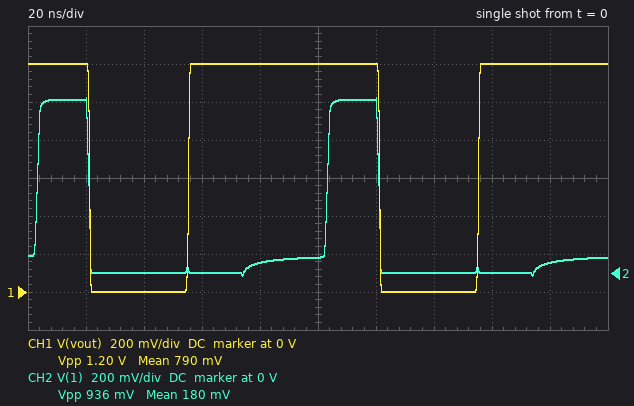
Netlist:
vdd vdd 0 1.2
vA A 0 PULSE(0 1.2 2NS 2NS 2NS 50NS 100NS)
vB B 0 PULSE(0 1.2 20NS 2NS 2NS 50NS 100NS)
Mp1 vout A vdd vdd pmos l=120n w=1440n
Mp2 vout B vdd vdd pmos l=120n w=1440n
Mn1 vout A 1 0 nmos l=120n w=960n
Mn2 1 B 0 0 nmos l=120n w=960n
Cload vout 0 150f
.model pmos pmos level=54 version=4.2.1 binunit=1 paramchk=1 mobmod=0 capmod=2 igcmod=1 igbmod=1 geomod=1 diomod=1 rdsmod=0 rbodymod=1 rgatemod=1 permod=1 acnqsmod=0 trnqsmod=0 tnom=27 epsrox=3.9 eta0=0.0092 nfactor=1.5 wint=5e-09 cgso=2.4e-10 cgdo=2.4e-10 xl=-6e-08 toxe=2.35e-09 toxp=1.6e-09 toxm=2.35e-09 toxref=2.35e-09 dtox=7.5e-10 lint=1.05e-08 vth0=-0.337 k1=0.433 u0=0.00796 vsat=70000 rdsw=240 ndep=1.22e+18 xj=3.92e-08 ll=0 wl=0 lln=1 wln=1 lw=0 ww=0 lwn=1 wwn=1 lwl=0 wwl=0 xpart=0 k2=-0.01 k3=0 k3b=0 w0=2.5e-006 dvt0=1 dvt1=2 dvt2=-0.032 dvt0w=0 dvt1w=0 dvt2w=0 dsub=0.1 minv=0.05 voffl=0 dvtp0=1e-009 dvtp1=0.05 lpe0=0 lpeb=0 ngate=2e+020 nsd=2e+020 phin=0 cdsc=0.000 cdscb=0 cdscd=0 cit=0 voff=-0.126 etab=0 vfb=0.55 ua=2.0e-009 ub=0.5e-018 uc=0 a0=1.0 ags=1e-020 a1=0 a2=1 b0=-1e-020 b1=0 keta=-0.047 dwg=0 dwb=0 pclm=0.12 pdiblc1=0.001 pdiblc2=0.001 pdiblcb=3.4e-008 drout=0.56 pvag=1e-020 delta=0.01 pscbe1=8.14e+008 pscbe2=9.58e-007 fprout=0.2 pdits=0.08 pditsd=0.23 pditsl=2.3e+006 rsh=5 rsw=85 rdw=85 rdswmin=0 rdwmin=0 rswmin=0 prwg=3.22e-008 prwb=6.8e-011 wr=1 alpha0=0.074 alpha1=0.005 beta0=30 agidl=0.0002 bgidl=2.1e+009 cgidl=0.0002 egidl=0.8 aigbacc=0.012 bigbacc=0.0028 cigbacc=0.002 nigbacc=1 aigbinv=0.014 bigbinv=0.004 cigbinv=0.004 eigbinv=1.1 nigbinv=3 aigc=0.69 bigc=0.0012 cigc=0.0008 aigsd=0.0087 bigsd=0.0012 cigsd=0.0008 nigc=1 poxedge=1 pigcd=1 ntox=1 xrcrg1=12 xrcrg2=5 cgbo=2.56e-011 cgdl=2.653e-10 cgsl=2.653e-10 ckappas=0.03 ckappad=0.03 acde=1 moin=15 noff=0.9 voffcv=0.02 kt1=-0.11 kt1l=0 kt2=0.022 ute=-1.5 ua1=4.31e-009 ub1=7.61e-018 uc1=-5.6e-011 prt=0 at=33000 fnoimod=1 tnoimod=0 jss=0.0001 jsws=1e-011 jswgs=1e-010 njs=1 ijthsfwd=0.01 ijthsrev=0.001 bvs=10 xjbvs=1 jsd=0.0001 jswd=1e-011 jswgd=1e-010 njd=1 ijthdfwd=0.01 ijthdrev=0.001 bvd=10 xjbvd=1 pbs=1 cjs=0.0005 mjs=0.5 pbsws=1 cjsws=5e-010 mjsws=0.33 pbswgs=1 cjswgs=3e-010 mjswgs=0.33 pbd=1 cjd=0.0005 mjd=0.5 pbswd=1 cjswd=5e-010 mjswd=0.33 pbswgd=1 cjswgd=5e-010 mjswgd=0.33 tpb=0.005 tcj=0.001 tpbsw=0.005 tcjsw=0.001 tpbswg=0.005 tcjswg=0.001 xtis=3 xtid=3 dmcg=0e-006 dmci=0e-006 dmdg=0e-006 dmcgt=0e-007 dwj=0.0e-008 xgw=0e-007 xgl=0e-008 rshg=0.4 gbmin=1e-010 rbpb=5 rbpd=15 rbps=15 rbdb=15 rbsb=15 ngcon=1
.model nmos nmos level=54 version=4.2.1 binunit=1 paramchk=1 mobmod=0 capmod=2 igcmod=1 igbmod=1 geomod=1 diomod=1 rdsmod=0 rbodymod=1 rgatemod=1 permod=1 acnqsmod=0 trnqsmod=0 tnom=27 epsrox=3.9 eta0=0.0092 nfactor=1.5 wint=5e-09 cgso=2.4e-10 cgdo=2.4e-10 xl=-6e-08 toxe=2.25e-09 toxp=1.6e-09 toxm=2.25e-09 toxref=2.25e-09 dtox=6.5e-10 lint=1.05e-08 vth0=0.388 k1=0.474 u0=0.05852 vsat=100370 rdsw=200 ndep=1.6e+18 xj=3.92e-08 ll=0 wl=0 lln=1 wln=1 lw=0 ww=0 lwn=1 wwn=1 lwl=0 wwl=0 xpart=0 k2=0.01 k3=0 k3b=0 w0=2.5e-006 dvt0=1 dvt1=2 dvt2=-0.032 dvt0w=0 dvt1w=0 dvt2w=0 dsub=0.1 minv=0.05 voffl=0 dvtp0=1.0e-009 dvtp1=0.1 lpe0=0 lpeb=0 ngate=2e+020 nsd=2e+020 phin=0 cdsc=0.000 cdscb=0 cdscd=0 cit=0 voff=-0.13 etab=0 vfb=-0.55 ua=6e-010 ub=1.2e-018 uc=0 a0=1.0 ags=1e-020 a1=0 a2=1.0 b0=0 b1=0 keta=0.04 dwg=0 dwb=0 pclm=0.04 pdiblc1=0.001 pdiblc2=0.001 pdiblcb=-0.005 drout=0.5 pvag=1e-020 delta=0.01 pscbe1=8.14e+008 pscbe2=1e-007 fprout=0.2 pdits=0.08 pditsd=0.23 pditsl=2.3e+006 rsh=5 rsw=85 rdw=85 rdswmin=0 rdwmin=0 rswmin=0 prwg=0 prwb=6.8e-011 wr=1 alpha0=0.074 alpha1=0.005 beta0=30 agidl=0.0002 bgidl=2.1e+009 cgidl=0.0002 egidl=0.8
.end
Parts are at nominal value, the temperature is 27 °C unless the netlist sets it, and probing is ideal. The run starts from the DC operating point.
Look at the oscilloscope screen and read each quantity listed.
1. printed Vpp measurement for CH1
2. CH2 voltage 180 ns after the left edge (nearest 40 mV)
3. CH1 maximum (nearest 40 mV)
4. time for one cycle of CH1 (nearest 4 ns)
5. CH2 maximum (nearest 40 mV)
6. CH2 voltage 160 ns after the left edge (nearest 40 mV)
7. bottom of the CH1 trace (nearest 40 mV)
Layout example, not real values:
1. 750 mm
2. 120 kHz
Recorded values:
1. 1.20 V
2. 40 mV
3. 1.20 V
4. 100 ns
5. 920 mV
6. 0 V
7. 0 V
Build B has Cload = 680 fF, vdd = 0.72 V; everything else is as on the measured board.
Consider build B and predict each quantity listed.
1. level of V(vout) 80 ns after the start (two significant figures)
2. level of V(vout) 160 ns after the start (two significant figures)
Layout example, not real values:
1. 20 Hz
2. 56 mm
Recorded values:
1. 720 mV
2. 710 mV
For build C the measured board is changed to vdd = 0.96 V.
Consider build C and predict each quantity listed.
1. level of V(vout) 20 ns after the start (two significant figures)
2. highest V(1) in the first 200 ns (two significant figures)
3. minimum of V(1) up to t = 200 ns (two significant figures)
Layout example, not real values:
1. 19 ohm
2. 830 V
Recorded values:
1. 960 mV
2. 900 mV
3. -23 mV
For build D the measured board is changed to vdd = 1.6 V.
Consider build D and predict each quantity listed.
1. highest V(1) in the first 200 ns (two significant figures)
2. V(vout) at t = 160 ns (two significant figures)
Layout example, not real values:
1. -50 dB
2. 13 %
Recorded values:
1. 950 mV
2. 1.6 V
